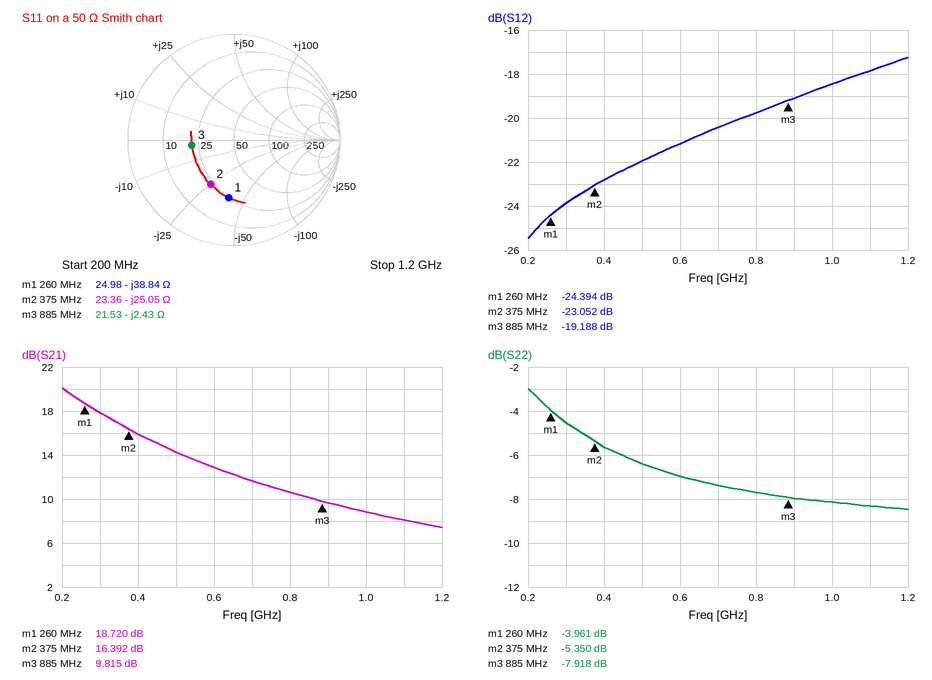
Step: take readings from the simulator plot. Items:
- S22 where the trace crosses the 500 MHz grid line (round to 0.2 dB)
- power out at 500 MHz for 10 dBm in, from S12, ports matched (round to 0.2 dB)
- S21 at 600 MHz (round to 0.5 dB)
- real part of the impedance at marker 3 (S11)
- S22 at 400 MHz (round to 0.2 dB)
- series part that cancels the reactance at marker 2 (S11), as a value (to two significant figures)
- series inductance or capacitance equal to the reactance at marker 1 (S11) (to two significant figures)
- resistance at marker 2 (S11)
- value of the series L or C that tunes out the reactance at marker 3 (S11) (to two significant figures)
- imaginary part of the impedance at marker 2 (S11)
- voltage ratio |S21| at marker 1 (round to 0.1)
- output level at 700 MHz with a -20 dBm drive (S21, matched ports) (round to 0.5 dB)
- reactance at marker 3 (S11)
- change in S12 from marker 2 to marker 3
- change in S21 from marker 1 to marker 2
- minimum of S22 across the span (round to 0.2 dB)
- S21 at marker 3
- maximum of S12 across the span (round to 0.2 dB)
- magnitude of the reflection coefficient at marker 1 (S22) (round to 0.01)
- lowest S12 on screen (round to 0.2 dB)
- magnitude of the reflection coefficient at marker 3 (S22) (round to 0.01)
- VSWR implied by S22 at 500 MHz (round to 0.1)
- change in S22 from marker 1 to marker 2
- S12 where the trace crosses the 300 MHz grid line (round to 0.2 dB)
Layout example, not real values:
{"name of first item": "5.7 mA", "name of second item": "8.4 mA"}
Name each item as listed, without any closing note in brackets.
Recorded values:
{"S22 where the trace crosses the 500 MHz grid line": "-6.4 dB", "power out at 500 MHz for 10 dBm in, from S12, ports matched": "-12.0 dBm", "S21 at 600 MHz": "13.0 dB", "real part of the impedance at marker 3": "21.53 Ω", "S22 at 400 MHz": "-5.6 dB", "series part that cancels the reactance at marker 2 (S11), as a value": "11 nH", "series inductance or capacitance equal to the reactance at marker 1 (S11)": "16 pF", "resistance at marker 2": "23.36 Ω", "value of the series L or C that tunes out the reactance at marker 3 (S11)": "440 pH", "imaginary part of the impedance at marker 2": "-25.05 Ω", "voltage ratio |S21| at marker 1": "8.6", "output level at 700 MHz with a -20 dBm drive (S21, matched ports)": "-8.5 dBm", "reactance at marker 3": "-2.43 Ω", "change in S12 from marker 2 to marker 3": "3.864 dB", "change in S21 from marker 1 to marker 2": "-2.328 dB", "minimum of S22 across the span": "-8.4 dB", "S21 at marker 3": "9.815 dB", "maximum of S12 across the span": "-17.2 dB", "magnitude of the reflection coefficient at marker 1 (S22)": "0.63", "lowest S12 on screen": "-25.4 dB", "magnitude of the reflection coefficient at marker 3 (S22)": "0.40", "VSWR implied by S22 at 500 MHz": "2.8", "change in S22 from marker 1 to marker 2": "-1.389 dB", "S12 where the trace crosses the 300 MHz grid line": "-23.8 dB"}
